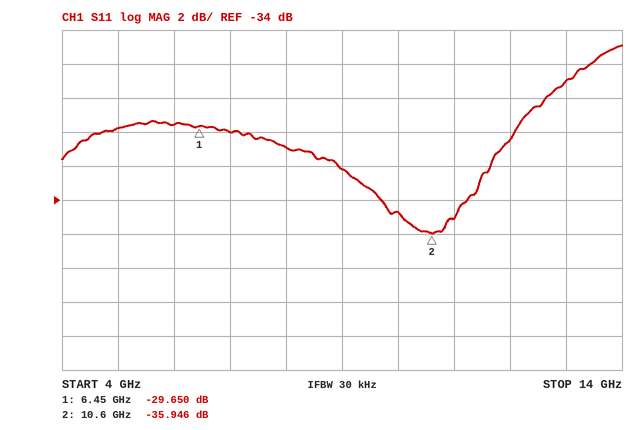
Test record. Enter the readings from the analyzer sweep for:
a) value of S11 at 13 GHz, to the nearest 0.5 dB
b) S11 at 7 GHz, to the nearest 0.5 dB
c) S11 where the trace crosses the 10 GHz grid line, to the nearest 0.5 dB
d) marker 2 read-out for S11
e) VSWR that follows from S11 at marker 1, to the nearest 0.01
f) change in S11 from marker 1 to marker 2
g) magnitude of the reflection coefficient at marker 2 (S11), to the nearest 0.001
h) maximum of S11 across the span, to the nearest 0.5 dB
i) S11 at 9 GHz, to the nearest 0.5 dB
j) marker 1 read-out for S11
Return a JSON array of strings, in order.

["-27.0 dB", "-30.0 dB", "-34.5 dB", "-35.946 dB", "1.07", "-6.296 dB", "0.016", "-25.0 dB", "-32.0 dB", "-29.650 dB"]
